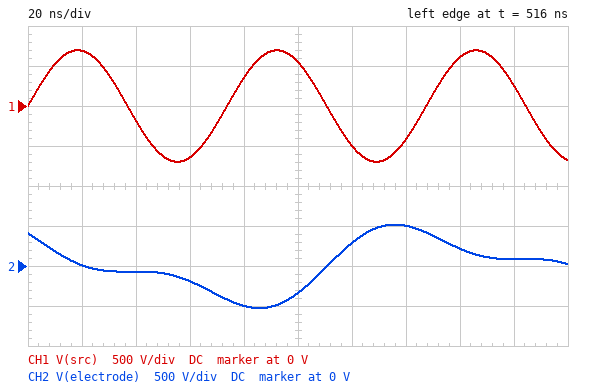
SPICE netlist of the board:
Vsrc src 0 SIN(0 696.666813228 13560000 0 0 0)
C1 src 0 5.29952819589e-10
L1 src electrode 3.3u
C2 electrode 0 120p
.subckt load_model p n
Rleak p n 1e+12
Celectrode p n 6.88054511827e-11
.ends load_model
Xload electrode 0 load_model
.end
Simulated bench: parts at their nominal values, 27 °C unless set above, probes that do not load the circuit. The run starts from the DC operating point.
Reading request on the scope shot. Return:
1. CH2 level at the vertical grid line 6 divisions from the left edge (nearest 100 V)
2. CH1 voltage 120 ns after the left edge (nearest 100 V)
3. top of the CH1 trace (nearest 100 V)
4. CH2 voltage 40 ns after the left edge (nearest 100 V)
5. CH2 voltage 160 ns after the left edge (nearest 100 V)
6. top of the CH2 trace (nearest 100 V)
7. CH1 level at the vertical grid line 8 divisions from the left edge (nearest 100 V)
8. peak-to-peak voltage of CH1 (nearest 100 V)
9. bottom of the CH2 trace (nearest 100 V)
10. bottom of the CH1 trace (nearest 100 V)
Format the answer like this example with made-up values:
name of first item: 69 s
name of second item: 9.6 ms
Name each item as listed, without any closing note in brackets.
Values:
CH2 level at the vertical grid line 6 divisions from the left edge: 300 V
CH1 voltage 120 ns after the left edge: -500 V
top of the CH1 trace: 700 V
CH2 voltage 40 ns after the left edge: -100 V
CH2 voltage 160 ns after the left edge: 200 V
top of the CH2 trace: 500 V
CH1 level at the vertical grid line 8 divisions from the left edge: 600 V
peak-to-peak voltage of CH1: 1.4 kV
bottom of the CH2 trace: -500 V
bottom of the CH1 trace: -700 V
